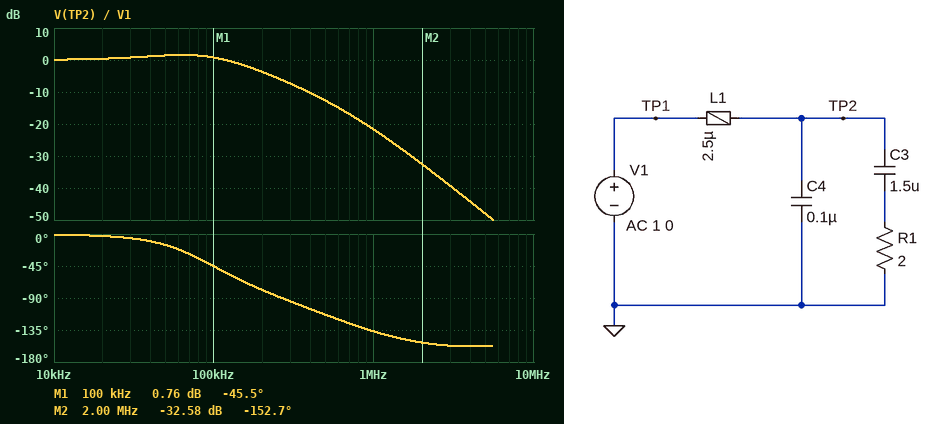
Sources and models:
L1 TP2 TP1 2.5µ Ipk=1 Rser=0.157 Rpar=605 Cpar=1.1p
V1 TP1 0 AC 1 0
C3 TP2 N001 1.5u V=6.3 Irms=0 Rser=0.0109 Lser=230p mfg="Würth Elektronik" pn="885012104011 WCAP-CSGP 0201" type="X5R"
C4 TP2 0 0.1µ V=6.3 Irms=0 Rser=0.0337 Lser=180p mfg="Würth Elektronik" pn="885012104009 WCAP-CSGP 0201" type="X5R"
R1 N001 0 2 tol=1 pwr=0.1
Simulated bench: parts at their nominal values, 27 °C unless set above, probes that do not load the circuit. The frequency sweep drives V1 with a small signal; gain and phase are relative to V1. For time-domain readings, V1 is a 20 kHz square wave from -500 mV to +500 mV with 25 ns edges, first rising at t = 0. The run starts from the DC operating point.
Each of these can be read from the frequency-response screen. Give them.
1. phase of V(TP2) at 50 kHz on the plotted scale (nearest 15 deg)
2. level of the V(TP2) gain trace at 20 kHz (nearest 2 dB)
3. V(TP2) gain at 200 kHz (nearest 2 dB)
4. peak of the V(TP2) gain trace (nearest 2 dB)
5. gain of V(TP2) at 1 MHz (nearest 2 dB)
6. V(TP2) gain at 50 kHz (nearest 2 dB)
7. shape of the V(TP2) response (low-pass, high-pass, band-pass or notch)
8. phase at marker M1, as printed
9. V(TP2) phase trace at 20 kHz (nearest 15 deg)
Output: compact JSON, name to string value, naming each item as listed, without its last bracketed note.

{"phase of V(TP2) at 50 kHz on the plotted scale": "-15 deg", "level of the V(TP2) gain trace at 20 kHz": "0 dB", "V(TP2) gain at 200 kHz": "-4 dB", "peak of the V(TP2) gain trace": "2 dB", "gain of V(TP2) at 1 MHz": "-22 dB", "V(TP2) gain at 50 kHz": "2 dB", "shape of the V(TP2) response": "low-pass", "phase at marker M1, as printed": "-45.5 deg", "V(TP2) phase trace at 20 kHz": "0 deg"}
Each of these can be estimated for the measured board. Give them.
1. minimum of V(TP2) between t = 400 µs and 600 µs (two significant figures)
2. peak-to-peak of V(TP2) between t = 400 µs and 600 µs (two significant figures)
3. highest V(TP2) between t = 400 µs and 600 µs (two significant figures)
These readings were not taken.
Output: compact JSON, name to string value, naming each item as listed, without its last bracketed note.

{"minimum of V(TP2) between t = 400 µs and 600 µs": "-670 mV", "peak-to-peak of V(TP2) between t = 400 µs and 600 µs": "1.3 V", "highest V(TP2) between t = 400 µs and 600 µs": "670 mV"}
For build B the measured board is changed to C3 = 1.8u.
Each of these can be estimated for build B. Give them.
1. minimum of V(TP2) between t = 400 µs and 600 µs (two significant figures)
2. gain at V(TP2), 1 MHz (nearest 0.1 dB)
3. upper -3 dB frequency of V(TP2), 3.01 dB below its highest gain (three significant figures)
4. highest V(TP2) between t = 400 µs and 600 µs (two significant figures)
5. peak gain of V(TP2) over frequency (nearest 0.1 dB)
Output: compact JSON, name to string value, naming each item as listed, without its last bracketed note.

{"minimum of V(TP2) between t = 400 µs and 600 µs": "-640 mV", "gain at V(TP2), 1 MHz": "-21.7 dB", "upper -3 dB frequency of V(TP2), 3.01 dB below its highest gain": "147 kHz", "highest V(TP2) between t = 400 µs and 600 µs": "640 mV", "peak gain of V(TP2) over frequency": "1.3 dB"}
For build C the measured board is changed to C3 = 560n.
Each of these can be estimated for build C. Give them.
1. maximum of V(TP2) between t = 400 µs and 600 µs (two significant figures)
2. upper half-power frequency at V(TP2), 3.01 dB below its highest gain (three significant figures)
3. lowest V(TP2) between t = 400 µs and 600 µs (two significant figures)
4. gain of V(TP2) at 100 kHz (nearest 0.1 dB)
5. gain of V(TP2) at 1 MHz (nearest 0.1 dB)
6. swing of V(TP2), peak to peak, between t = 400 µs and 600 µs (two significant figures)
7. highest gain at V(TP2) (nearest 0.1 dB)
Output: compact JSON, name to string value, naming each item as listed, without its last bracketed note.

{"maximum of V(TP2) between t = 400 µs and 600 µs": "860 mV", "upper half-power frequency at V(TP2), 3.01 dB below its highest gain": "173 kHz", "lowest V(TP2) between t = 400 µs and 600 µs": "-860 mV", "gain of V(TP2) at 100 kHz": "3.9 dB", "gain of V(TP2) at 1 MHz": "-22.1 dB", "swing of V(TP2), peak to peak, between t = 400 µs and 600 µs": "1.7 V", "highest gain at V(TP2)": "4.2 dB"}
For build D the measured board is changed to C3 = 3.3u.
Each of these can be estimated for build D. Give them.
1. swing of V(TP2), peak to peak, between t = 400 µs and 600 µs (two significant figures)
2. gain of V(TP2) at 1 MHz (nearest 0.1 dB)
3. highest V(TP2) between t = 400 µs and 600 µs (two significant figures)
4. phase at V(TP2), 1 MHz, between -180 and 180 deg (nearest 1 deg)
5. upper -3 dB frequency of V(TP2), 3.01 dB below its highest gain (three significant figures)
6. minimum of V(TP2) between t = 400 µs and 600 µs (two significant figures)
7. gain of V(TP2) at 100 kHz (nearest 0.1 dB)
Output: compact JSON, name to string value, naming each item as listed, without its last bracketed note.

{"swing of V(TP2), peak to peak, between t = 400 µs and 600 µs": "1.1 V", "gain of V(TP2) at 1 MHz": "-21.7 dB", "highest V(TP2) between t = 400 µs and 600 µs": "560 mV", "phase at V(TP2), 1 MHz, between -180 and 180 deg": "-136 deg", "upper -3 dB frequency of V(TP2), 3.01 dB below its highest gain": "146 kHz", "minimum of V(TP2) between t = 400 µs and 600 µs": "-560 mV", "gain of V(TP2) at 100 kHz": "-0.9 dB"}
